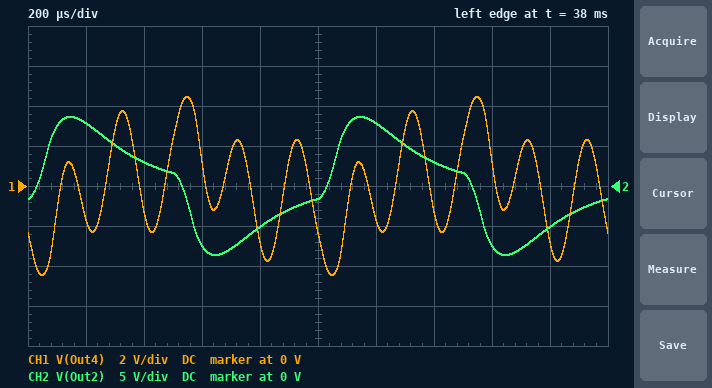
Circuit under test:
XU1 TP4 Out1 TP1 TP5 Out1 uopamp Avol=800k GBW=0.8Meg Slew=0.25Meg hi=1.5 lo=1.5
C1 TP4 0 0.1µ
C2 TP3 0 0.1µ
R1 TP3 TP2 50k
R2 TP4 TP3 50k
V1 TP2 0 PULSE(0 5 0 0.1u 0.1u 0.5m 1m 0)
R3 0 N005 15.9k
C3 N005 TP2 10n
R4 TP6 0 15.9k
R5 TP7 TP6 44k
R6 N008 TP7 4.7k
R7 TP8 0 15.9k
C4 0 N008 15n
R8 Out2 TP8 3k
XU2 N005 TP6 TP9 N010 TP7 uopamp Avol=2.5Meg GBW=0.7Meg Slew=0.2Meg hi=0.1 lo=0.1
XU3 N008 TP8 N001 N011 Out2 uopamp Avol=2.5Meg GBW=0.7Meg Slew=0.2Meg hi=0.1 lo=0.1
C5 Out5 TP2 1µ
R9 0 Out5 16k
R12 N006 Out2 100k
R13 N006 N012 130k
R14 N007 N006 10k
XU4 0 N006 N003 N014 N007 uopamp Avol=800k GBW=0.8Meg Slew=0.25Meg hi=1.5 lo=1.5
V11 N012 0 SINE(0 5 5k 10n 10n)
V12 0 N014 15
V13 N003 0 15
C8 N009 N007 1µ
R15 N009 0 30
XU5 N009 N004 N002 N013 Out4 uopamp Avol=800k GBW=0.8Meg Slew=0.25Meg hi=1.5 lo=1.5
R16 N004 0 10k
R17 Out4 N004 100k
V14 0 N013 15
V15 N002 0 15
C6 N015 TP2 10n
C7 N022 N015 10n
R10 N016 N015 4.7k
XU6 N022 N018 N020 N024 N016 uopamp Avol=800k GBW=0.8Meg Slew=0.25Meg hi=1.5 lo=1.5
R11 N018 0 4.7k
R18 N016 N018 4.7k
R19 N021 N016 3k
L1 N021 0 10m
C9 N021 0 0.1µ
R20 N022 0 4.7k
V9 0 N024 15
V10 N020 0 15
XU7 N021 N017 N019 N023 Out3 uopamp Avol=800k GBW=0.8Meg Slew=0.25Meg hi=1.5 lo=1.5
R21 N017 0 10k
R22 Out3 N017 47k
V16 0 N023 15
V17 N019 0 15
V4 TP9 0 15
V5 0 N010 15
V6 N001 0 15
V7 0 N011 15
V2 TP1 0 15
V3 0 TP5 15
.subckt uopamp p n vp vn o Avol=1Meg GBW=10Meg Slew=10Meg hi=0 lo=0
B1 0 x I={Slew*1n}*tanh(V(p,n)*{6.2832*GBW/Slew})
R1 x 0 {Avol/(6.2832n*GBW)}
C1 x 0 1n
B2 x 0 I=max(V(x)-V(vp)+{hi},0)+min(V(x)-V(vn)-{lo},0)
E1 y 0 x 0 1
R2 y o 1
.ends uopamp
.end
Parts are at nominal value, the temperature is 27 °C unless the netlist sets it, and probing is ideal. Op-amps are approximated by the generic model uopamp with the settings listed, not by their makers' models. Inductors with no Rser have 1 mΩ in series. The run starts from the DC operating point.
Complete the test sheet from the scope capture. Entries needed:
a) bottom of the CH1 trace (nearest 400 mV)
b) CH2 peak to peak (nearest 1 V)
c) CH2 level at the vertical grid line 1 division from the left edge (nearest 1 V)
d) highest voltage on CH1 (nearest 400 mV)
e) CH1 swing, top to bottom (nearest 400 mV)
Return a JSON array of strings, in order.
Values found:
["-4.4 V", "17 V", "8 V", "4.4 V", "8.8 V"]
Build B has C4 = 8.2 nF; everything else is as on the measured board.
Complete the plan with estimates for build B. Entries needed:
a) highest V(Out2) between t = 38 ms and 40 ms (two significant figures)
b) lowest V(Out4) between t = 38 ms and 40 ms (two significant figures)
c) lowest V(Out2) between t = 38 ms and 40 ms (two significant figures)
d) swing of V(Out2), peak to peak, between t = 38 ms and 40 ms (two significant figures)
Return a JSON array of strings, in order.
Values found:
["11 V", "-5.5 V", "-11 V", "21 V"]
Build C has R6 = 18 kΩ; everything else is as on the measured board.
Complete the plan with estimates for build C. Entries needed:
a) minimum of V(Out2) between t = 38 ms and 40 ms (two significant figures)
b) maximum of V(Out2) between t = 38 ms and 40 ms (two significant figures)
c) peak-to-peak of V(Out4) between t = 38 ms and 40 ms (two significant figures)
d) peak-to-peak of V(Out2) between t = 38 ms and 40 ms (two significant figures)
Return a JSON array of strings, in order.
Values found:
["-3.7 V", "3.7 V", "6.7 V", "7.4 V"]
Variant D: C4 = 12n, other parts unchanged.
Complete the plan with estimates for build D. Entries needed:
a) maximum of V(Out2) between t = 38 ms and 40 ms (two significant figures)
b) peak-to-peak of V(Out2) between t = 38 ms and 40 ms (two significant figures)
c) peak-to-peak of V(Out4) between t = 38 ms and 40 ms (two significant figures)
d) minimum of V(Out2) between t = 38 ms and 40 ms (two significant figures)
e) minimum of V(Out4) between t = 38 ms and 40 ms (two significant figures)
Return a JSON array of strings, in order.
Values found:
["9.4 V", "19 V", "9.6 V", "-9.4 V", "-4.8 V"]
